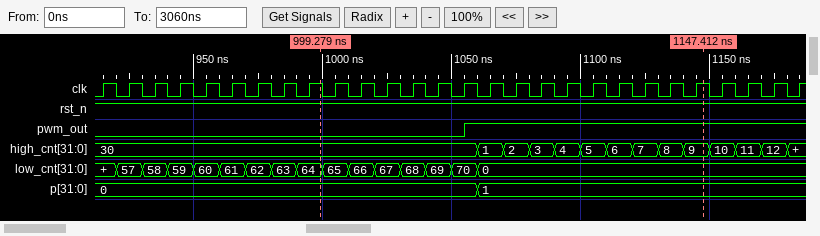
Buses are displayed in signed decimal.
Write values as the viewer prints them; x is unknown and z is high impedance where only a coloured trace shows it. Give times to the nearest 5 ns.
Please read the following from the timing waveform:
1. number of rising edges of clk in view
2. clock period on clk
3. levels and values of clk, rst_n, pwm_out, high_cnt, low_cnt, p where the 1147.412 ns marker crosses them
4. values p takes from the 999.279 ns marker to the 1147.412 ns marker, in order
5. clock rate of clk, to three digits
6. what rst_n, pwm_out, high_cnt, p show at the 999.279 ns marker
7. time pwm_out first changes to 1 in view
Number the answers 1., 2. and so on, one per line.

1. 28
2. 10 ns
3. clk=1, rst_n=1, pwm_out=1, high_cnt=9, low_cnt=0, p=1
4. 0, 1
5. 100 MHz
6. rst_n=1, pwm_out=0, high_cnt=30, p=0
7. 1055 ns
